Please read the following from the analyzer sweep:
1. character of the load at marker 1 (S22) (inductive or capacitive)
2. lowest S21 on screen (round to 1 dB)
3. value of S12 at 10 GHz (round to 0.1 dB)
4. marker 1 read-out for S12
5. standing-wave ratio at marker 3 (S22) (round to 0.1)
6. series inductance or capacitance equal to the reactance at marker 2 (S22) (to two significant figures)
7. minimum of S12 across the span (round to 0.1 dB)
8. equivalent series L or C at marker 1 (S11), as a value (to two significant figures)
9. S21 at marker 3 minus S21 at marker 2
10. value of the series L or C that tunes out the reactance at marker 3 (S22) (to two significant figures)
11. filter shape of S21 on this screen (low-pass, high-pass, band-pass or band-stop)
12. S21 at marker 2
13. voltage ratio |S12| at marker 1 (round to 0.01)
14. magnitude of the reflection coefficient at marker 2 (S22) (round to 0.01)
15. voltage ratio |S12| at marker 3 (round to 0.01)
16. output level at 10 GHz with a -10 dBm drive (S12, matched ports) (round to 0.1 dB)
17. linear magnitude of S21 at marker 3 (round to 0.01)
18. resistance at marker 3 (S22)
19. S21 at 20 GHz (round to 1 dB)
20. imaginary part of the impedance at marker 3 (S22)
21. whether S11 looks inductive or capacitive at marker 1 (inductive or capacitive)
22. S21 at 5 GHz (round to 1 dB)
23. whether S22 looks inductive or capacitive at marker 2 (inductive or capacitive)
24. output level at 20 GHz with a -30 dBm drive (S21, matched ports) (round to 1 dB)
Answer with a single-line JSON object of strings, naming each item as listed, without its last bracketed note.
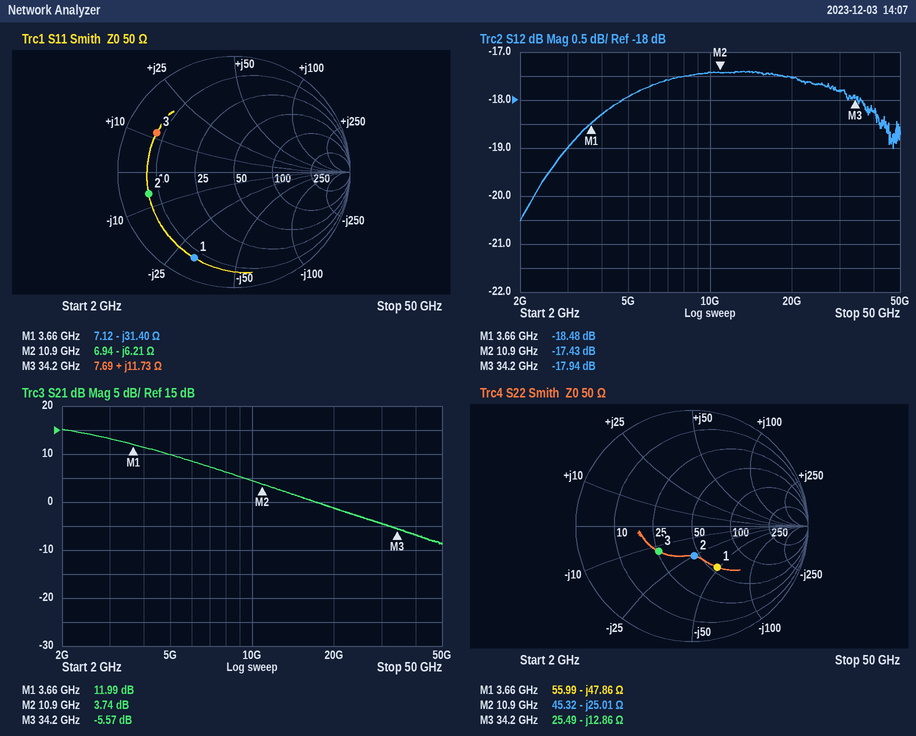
{"character of the load at marker 1 (S22)": "capacitive", "lowest S21 on screen": "-9 dB", "value of S12 at 10 GHz": "-17.4 dB", "marker 1 read-out for S12": "-18.48 dB", "standing-wave ratio at marker 3 (S22)": "2.1", "series inductance or capacitance equal to the reactance at marker 2 (S22)": "580 fF", "minimum of S12 across the span": "-20.5 dB", "equivalent series L or C at marker 1 (S11), as a value": "1.4 pF", "S21 at marker 3 minus S21 at marker 2": "-9.31 dB", "value of the series L or C that tunes out the reactance at marker 3 (S22)": "60 pH", "filter shape of S21 on this screen": "low-pass", "S21 at marker 2": "3.74 dB", "voltage ratio |S12| at marker 1": "0.12", "magnitude of the reflection coefficient at marker 2 (S22)": "0.26", "voltage ratio |S12| at marker 3": "0.13", "output level at 10 GHz with a -10 dBm drive (S12, matched ports)": "-27.4 dBm", "linear magnitude of S21 at marker 3": "0.53", "resistance at marker 3": "25.49 Ω", "S21 at 20 GHz": "-1 dB", "imaginary part of the impedance at marker 3": "-12.86 Ω", "whether S11 looks inductive or capacitive at marker 1": "capacitive", "S21 at 5 GHz": "10 dB", "whether S22 looks inductive or capacitive at marker 2": "capacitive", "output level at 20 GHz with a -30 dBm drive (S21, matched ports)": "-31 dBm"}
